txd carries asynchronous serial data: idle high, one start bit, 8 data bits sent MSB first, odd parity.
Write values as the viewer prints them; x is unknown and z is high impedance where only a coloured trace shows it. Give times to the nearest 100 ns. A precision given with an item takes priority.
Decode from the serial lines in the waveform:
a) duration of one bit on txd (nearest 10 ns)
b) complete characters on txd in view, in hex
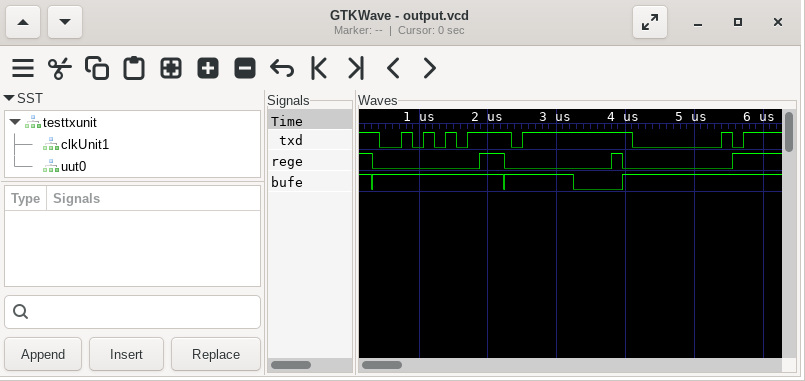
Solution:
160 ns
55, FF, 01
